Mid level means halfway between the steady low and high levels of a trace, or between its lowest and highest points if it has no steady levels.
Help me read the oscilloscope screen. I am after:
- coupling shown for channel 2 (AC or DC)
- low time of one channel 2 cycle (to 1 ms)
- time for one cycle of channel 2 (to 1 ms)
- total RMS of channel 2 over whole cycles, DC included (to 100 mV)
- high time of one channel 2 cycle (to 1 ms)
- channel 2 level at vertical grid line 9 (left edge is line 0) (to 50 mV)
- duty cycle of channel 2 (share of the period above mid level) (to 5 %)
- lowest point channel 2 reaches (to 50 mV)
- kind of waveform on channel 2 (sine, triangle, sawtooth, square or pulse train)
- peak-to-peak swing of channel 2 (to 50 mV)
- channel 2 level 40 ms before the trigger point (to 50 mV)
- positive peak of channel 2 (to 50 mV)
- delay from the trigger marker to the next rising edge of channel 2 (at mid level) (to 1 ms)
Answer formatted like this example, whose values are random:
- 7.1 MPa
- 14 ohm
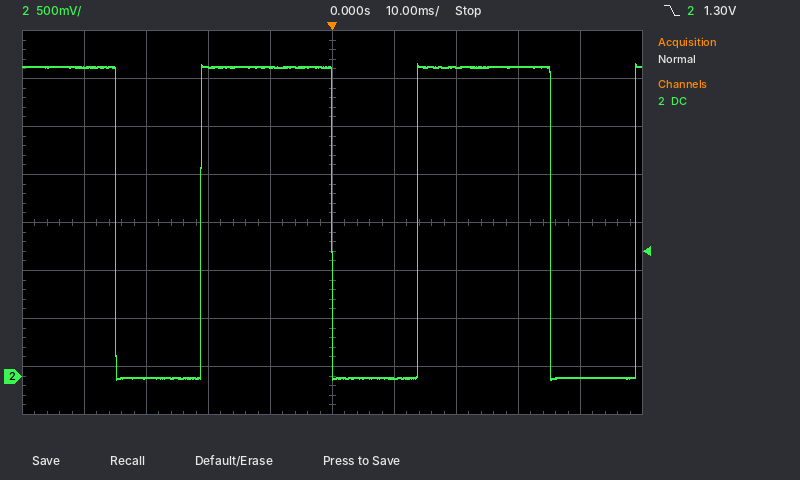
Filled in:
- DC
- 14 ms
- 35 ms
- 2.5 V
- 21 ms
- 0 mV
- 60 %
- -50 mV
- pulse train
- 3.30 V
- 3.20 V
- 3.25 V
- 14 ms
